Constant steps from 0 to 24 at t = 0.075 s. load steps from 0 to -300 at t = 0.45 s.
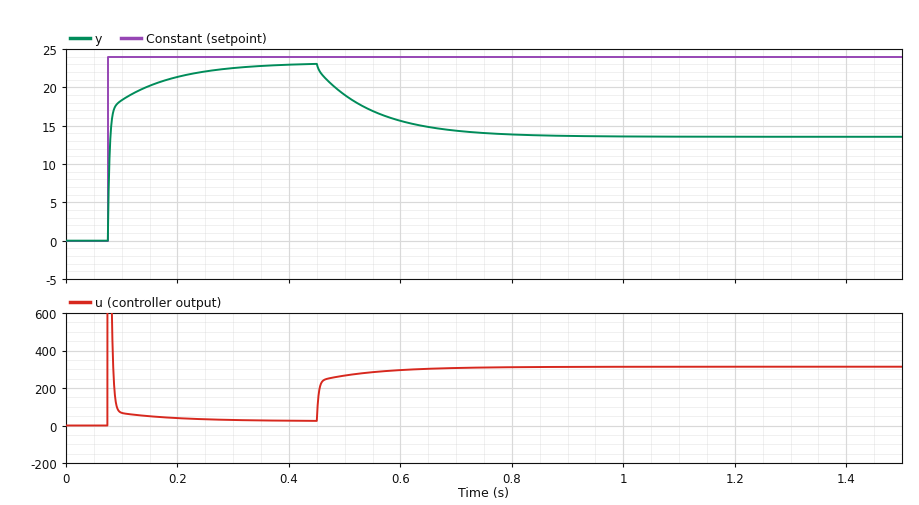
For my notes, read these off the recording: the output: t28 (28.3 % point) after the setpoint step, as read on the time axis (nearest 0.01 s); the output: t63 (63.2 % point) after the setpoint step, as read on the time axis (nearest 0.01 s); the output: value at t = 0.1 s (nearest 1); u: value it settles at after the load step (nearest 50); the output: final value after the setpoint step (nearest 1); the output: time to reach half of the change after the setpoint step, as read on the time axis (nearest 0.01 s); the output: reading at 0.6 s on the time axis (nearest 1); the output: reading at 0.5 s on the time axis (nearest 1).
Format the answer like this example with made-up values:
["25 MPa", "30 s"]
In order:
["0.08 s", "0.08 s", "18", "300", "23", "0.08 s", "16", "19"]
